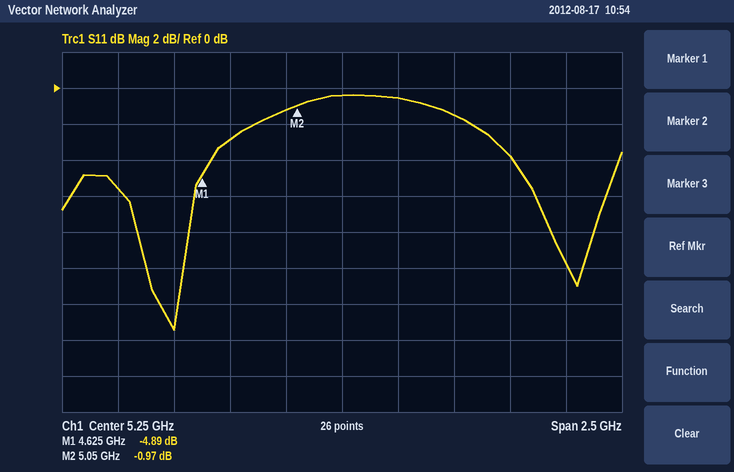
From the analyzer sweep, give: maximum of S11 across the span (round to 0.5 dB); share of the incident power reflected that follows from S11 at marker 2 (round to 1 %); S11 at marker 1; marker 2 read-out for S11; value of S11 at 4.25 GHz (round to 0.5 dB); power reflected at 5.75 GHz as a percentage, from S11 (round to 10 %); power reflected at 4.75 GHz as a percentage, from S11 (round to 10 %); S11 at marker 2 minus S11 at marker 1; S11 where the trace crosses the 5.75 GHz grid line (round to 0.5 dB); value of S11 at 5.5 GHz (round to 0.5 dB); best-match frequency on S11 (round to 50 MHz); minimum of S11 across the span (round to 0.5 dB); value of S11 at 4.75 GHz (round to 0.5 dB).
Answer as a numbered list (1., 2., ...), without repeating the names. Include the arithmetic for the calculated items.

1. -0.5 dB
2. 10^(-0.97/10) ≈ 80 %
3. -4.89 dB
4. -0.97 dB
5. -5.5 dB
6. 10^(-1.5/10) ≈ 70.8 %, so 70 % to the nearest 10 %
7. 10^(-3/10) ≈ 50 %
8. -0.97 − (-4.89) = 3.92 dB
9. -1.5 dB
10. -0.5 dB
11. 4.50 GHz
12. -13.5 dB
13. -3.0 dB
